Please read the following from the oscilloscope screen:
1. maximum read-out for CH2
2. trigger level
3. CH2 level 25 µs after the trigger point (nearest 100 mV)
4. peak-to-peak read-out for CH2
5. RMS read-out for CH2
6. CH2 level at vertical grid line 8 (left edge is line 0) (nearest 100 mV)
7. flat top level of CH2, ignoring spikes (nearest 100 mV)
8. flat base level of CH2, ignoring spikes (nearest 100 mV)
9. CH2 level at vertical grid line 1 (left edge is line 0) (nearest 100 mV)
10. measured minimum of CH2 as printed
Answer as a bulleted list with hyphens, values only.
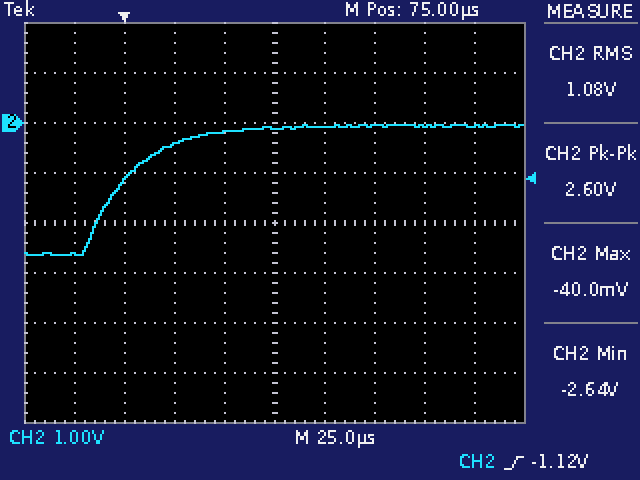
- -40.0 mV
- -1.12 V
- -400 mV
- 2.60 V
- 1.08 V
- -100 mV
- -100 mV
- -2.6 V
- -2.6 V
- -2.64 V
